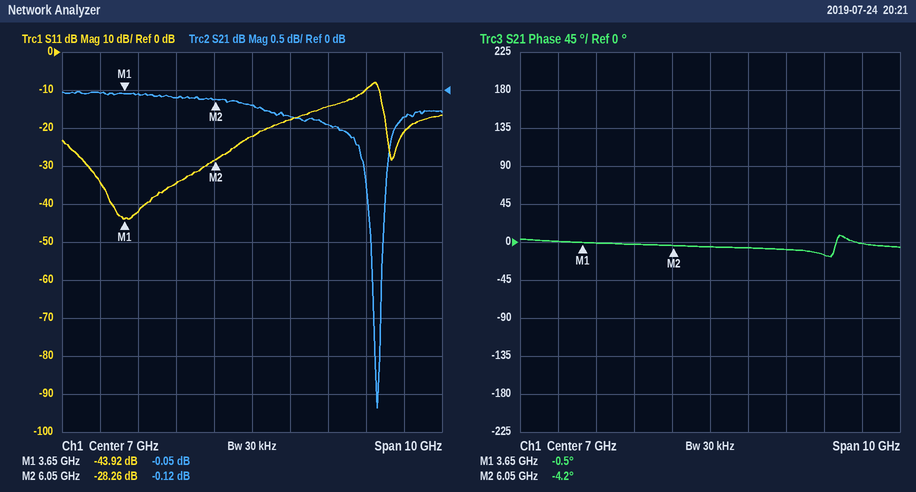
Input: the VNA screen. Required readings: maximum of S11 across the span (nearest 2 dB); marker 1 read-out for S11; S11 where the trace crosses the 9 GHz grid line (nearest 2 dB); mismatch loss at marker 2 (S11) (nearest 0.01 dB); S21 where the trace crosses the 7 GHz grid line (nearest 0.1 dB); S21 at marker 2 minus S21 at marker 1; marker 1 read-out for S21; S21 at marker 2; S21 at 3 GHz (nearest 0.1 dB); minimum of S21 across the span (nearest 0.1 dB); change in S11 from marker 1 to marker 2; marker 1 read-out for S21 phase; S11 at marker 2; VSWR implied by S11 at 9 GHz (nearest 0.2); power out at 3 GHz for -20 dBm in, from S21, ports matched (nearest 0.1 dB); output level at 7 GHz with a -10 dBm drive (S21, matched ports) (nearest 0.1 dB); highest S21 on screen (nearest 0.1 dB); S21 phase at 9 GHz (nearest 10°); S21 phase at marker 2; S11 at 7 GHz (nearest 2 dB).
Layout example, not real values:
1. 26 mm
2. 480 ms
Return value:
1. -8 dB
2. -43.92 dB
3. -14 dB
4. 0.01 dB
5. -0.2 dB
6. -0.07 dB
7. -0.05 dB
8. -0.12 dB
9. 0.0 dB
10. -4.2 dB
11. 15.66 dB
12. -0.5°
13. -28.26 dB
14. 1.4
15. -20.0 dBm
16. -10.2 dBm
17. 0.0 dB
18. -10°
19. -4.2°
20. -22 dB
